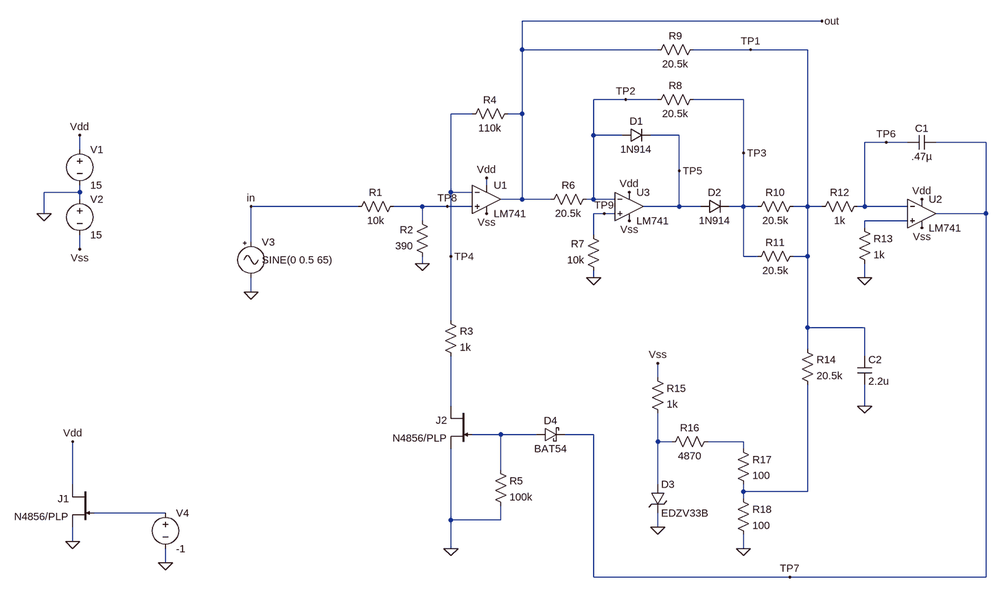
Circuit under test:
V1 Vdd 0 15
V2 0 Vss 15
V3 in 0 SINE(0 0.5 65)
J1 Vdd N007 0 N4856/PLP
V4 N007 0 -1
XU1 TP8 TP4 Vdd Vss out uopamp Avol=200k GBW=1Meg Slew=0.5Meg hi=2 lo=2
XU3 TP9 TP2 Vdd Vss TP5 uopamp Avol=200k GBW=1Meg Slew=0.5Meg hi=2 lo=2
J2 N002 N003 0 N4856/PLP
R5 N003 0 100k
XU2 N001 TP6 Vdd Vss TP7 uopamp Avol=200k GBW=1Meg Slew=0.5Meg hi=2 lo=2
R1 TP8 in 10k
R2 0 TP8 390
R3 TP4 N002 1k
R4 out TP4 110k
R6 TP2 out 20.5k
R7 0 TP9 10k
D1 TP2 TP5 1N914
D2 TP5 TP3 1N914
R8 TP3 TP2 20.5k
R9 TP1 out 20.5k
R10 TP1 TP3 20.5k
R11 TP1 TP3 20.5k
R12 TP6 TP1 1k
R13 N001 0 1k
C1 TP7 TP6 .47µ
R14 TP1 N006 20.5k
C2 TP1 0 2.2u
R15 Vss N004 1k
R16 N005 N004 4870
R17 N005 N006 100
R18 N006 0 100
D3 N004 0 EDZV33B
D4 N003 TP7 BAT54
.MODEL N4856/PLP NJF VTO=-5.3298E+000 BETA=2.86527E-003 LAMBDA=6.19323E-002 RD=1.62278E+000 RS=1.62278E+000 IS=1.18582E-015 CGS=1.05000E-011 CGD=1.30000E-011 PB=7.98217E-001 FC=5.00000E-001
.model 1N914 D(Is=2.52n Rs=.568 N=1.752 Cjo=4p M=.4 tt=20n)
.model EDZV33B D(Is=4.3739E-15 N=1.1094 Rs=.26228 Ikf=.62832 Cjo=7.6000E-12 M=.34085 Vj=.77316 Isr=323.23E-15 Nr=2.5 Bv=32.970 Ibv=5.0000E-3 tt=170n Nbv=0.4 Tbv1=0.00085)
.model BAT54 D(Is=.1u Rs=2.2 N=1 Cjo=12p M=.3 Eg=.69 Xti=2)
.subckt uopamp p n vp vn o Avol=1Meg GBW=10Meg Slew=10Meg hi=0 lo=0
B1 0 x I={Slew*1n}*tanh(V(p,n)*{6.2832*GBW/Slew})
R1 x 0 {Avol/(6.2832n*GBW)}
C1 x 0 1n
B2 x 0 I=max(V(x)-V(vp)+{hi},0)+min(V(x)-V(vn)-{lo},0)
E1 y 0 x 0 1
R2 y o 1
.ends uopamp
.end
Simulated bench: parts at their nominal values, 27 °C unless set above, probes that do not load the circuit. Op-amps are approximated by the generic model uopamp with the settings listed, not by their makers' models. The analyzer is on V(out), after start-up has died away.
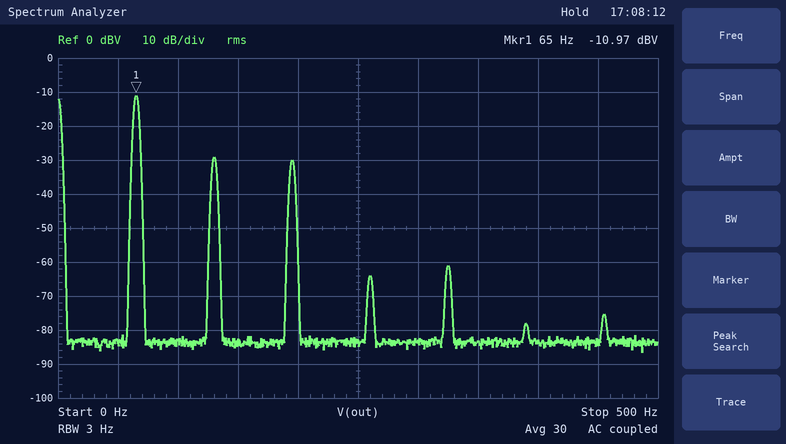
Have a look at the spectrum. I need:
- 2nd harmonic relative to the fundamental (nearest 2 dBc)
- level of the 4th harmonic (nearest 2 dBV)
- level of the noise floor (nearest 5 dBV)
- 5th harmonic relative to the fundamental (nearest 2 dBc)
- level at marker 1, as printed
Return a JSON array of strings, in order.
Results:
["-18 dBc", "-64 dBV", "-85 dBV", "-50 dBc", "-10.97 dBV"]
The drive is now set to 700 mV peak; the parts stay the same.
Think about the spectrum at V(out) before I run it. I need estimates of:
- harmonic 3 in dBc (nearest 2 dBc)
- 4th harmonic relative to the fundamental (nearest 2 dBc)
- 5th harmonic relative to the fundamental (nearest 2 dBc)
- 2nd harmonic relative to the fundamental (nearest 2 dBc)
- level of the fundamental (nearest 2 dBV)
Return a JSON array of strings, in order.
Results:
["-14 dBc", "-46 dBc", "-56 dBc", "-12 dBc", "-10 dBV"]
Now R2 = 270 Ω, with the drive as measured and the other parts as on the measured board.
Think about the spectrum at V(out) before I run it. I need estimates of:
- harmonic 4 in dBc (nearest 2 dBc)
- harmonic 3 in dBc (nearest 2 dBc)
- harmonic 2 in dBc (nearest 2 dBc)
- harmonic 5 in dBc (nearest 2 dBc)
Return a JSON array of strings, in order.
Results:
["-56 dBc", "-24 dBc", "-28 dBc", "-52 dBc"]
